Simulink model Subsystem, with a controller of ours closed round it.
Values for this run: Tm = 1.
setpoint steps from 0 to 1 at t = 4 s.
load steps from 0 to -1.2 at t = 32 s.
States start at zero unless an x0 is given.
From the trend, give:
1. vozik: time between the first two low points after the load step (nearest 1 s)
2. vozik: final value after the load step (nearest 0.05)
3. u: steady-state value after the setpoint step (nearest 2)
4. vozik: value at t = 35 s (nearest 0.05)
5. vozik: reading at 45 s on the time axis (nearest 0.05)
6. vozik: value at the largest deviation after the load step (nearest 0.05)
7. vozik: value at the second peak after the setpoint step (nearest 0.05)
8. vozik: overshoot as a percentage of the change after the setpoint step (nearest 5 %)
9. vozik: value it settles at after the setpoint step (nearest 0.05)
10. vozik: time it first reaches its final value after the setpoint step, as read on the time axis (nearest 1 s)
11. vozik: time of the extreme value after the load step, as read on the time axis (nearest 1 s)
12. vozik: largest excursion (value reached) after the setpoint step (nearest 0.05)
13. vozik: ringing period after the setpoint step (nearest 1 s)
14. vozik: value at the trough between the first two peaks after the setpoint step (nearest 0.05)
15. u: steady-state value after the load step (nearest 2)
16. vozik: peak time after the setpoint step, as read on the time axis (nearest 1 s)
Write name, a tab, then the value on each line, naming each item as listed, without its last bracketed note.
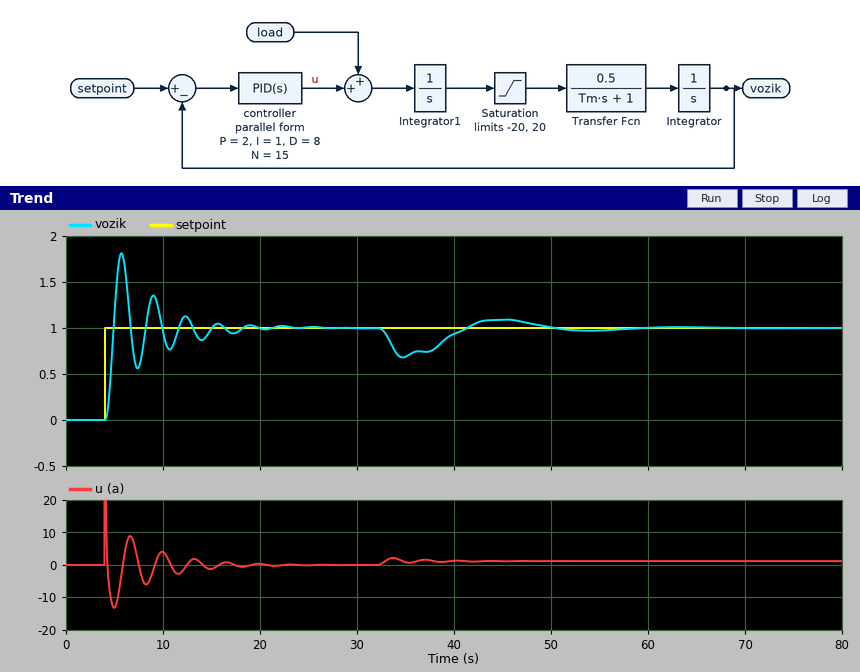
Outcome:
vozik: time between the first two low points after the load step	19 s
vozik: final value after the load step	1.00
u: steady-state value after the setpoint step	0
vozik: value at t = 35 s	0.70
vozik: reading at 45 s on the time axis	1.10
vozik: value at the largest deviation after the load step	0.70
vozik: value at the second peak after the setpoint step	1.35
vozik: overshoot as a percentage of the change after the setpoint step	80 %
vozik: value it settles at after the setpoint step	1.00
vozik: time it first reaches its final value after the setpoint step, as read on the time axis	5 s
vozik: time of the extreme value after the load step, as read on the time axis	35 s
vozik: largest excursion (value reached) after the setpoint step	1.80
vozik: ringing period after the setpoint step	3 s
vozik: value at the trough between the first two peaks after the setpoint step	0.55
u: steady-state value after the load step	2
vozik: peak time after the setpoint step, as read on the time axis	6 s
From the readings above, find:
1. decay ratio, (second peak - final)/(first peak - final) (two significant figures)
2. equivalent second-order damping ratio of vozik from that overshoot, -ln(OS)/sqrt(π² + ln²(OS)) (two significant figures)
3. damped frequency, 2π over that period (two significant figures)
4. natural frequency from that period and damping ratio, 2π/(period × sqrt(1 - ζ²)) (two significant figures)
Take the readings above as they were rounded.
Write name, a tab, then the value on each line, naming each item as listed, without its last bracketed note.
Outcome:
decay ratio, (second peak - final)/(first peak - final)	0.44
equivalent second-order damping ratio of vozik from that overshoot, -ln(OS)/sqrt(π² + ln²(OS))	0.071
damped frequency, 2π over that period	2.1 rad/s
natural frequency from that period and damping ratio, 2π/(period × sqrt(1 - ζ²))	2.1 rad/s
